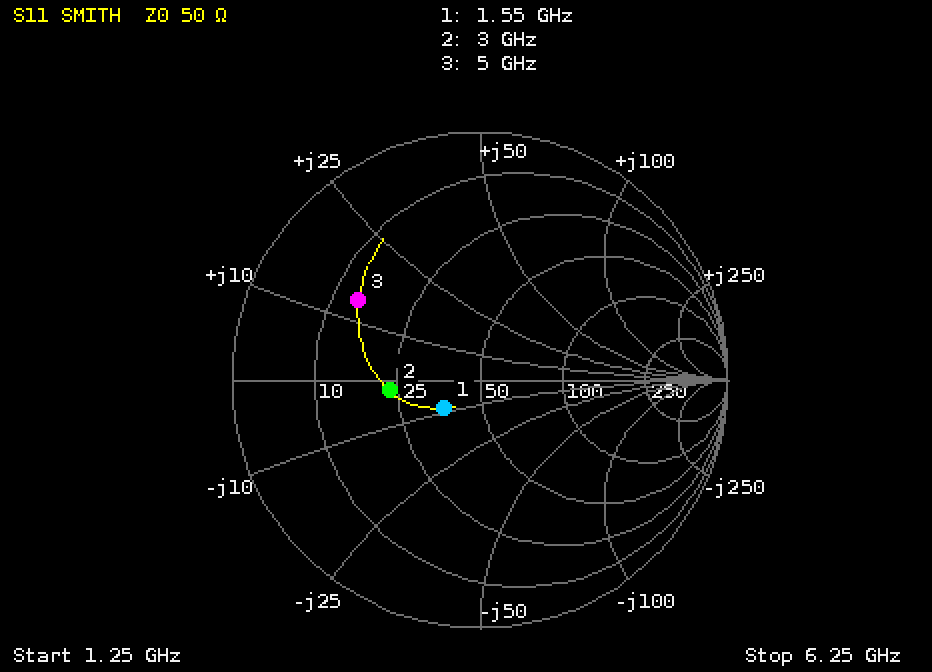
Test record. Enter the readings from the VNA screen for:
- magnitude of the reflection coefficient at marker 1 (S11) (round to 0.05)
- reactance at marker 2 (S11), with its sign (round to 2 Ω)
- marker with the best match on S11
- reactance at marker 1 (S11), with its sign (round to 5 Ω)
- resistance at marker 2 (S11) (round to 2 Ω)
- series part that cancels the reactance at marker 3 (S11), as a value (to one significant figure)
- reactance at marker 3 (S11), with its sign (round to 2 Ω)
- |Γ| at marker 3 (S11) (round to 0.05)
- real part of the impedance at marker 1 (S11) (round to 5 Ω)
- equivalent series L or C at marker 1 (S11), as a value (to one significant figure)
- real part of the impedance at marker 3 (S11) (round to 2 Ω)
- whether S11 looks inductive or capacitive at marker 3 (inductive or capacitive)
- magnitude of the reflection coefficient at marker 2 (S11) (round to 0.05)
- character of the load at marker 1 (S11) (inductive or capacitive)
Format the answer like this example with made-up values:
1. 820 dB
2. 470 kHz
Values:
1. 0.20
2. -2 Ω
3. marker 1
4. -10 Ω
5. 24 Ω
6. 2 pF
7. +14 Ω
8. 0.60
9. 35 Ω
10. 10 pF
11. 14 Ω
12. inductive
13. 0.35
14. capacitive
